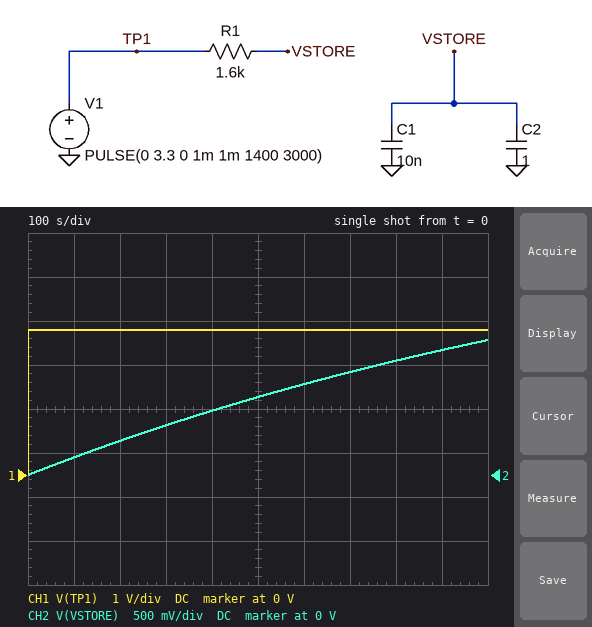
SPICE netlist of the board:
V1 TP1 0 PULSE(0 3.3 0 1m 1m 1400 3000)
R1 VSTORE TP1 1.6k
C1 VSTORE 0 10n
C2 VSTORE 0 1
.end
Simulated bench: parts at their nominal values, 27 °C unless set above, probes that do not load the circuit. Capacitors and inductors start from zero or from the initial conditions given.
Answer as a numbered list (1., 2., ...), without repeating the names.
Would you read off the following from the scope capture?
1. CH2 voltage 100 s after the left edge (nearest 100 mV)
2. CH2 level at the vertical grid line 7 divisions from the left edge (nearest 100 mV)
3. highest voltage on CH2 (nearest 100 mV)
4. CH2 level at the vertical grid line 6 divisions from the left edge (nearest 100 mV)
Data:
1. 200 mV
2. 1.2 V
3. 1.5 V
4. 1.0 V
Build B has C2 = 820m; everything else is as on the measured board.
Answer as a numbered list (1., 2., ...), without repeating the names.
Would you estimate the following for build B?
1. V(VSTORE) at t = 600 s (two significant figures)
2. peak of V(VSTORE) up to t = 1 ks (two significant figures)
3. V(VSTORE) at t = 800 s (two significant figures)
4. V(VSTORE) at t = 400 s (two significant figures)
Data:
1. 1.2 V
2. 1.8 V
3. 1.5 V
4. 870 mV
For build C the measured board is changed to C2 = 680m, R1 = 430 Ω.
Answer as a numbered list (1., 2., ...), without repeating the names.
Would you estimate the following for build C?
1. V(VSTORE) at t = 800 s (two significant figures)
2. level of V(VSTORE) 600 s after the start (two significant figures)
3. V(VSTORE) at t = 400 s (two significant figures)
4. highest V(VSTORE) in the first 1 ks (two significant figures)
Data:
1. 3.1 V
2. 2.9 V
3. 2.5 V
4. 3.2 V
